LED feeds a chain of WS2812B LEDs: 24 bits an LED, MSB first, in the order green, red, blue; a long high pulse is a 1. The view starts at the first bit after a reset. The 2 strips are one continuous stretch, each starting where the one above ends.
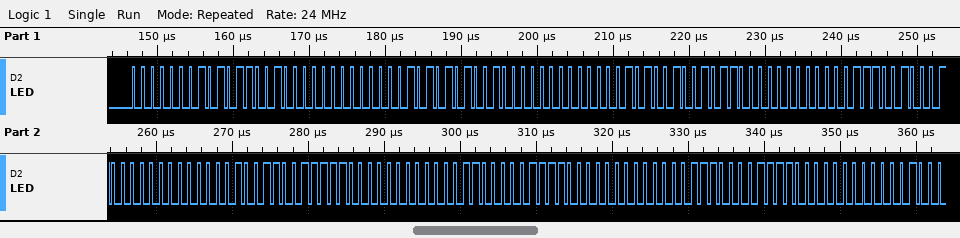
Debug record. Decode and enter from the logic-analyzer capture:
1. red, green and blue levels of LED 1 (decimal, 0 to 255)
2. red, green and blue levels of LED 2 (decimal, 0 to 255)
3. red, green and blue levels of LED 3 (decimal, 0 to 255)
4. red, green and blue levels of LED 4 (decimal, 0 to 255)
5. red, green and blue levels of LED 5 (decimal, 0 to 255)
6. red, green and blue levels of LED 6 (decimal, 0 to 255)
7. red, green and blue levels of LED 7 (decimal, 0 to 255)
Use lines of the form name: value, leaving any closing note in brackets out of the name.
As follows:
red, green and blue levels of LED 1: 89, 1, 0
red, green and blue levels of LED 2: 82, 5, 0
red, green and blue levels of LED 3: 75, 10, 0
red, green and blue levels of LED 4: 68, 14, 0
red, green and blue levels of LED 5: 62, 19, 0
red, green and blue levels of LED 6: 60, 24, 0
red, green and blue levels of LED 7: 60, 28, 0
